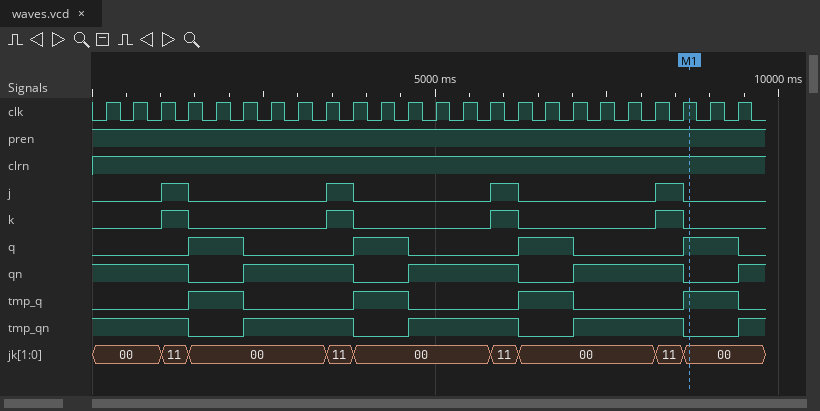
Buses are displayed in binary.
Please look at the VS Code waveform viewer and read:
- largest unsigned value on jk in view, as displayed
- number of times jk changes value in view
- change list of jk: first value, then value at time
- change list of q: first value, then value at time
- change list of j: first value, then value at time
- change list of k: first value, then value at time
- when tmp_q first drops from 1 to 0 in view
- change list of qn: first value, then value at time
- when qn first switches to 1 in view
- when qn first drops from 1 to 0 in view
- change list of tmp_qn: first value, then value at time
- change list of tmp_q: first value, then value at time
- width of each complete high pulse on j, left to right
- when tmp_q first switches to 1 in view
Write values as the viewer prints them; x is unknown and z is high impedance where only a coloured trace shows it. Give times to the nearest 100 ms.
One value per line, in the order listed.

11
8
00, 11 at 1000 ms, 00 at 1400 ms, 11 at 3400 ms, 00 at 3800 ms, 11 at 5800 ms, 00 at 6200 ms, 11 at 8200 ms, 00 at 8600 ms
0, 1 at 1400 ms, 0 at 2200 ms, 1 at 3800 ms, 0 at 4600 ms, 1 at 6200 ms, 0 at 7000 ms, 1 at 8600 ms, 0 at 9400 ms
0, 1 at 1000 ms, 0 at 1400 ms, 1 at 3400 ms, 0 at 3800 ms, 1 at 5800 ms, 0 at 6200 ms, 1 at 8200 ms, 0 at 8600 ms
0, 1 at 1000 ms, 0 at 1400 ms, 1 at 3400 ms, 0 at 3800 ms, 1 at 5800 ms, 0 at 6200 ms, 1 at 8200 ms, 0 at 8600 ms
2200 ms
1, 0 at 1400 ms, 1 at 2200 ms, 0 at 3800 ms, 1 at 4600 ms, 0 at 6200 ms, 1 at 7000 ms, 0 at 8600 ms, 1 at 9400 ms
2200 ms
1400 ms
1, 0 at 1400 ms, 1 at 2200 ms, 0 at 3800 ms, 1 at 4600 ms, 0 at 6200 ms, 1 at 7000 ms, 0 at 8600 ms, 1 at 9400 ms
0, 1 at 1400 ms, 0 at 2200 ms, 1 at 3800 ms, 0 at 4600 ms, 1 at 6200 ms, 0 at 7000 ms, 1 at 8600 ms, 0 at 9400 ms
400 ms, 400 ms, 400 ms, 400 ms
1400 ms
